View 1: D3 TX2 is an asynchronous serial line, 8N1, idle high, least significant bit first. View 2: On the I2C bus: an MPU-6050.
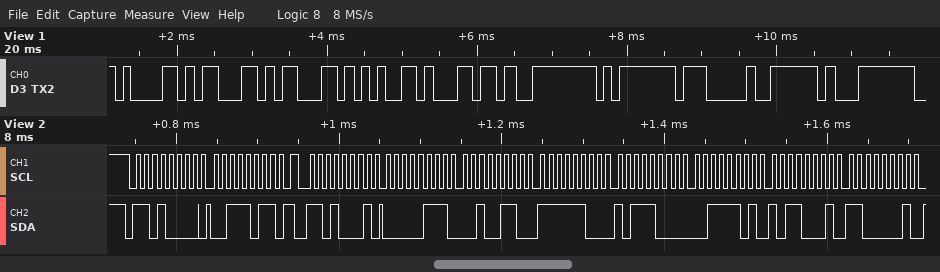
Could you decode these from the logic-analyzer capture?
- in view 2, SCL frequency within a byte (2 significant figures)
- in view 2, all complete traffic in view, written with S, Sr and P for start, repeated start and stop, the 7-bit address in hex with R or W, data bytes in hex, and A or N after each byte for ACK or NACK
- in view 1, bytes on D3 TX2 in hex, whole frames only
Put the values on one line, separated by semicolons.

100 kHz; S 68W A 3B A Sr 68R A 07 A 26 A FC A B8 A 3D A B1 A C1 A; 0x61 0x63 0x63 0x65 0x6C 0xFE 0xFD 0x07 0x7E 0xFC
